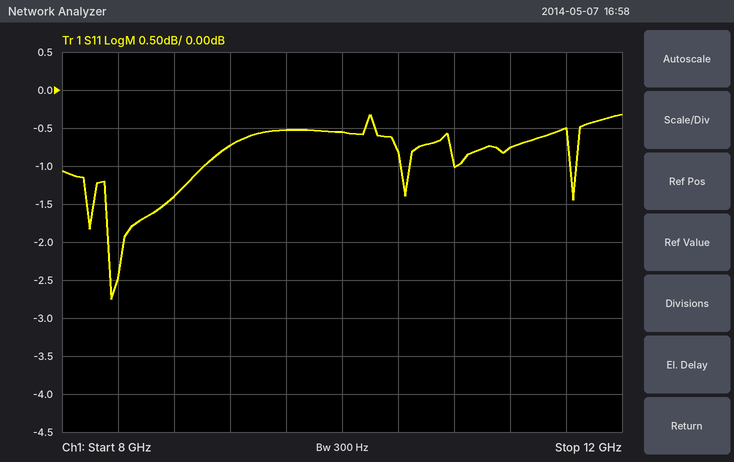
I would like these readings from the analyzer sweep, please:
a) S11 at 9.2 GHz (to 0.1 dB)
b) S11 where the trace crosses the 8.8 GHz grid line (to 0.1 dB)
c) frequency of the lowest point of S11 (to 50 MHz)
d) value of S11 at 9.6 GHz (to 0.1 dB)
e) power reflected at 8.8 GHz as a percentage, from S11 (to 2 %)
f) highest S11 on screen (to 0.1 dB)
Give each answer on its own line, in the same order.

-0.7 dB
-1.4 dB
8.35 GHz
-0.5 dB
72 %
-0.3 dB
